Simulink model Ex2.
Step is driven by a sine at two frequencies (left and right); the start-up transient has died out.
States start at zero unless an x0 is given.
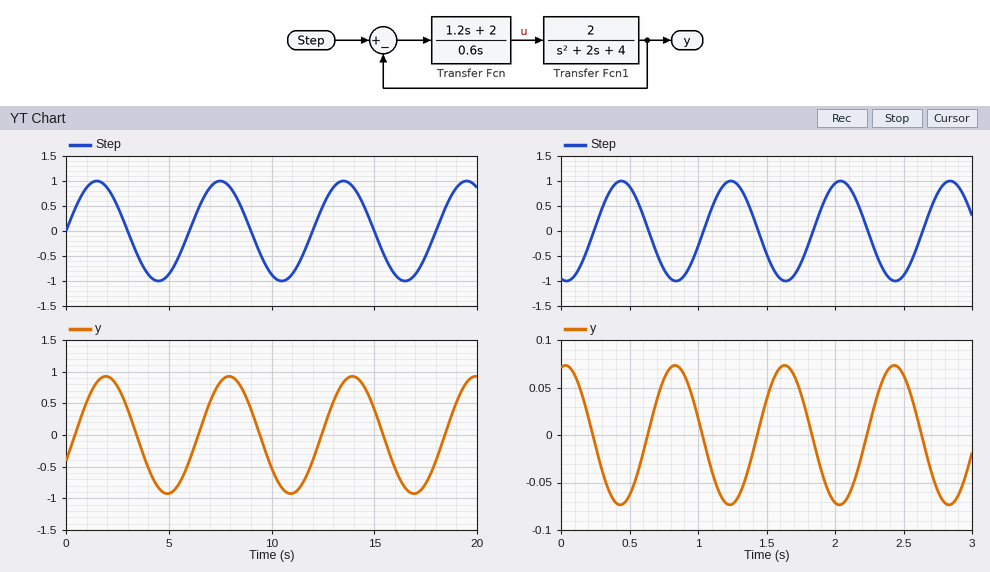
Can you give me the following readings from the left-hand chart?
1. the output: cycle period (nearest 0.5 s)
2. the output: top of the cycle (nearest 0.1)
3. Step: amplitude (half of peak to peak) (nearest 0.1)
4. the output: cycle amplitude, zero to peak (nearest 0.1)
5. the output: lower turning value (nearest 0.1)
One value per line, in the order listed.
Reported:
6.0 s
0.9
1.0
0.9
-0.9
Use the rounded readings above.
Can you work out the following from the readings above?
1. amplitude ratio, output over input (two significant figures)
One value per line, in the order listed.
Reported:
0.90
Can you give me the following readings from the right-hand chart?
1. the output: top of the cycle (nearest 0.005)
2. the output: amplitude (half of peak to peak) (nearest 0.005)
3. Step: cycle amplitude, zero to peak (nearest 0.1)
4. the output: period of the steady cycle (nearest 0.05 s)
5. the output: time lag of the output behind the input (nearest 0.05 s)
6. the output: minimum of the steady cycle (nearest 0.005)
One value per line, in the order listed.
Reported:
0.075
0.075
1.0
0.80 s
0.40 s
-0.075
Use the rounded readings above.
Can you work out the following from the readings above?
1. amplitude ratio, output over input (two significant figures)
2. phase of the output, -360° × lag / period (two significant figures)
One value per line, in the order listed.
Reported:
0.075
-180°
